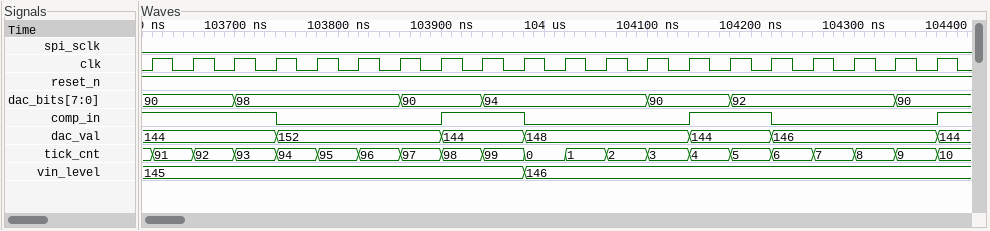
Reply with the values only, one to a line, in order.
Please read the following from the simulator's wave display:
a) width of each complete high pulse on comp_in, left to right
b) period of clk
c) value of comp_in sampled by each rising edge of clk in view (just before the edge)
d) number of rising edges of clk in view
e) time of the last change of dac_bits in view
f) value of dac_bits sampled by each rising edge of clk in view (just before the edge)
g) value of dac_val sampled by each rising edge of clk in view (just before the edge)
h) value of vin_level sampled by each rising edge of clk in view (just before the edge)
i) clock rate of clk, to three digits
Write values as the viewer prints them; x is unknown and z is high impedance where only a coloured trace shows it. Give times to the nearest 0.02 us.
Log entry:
0.08 us, 0.08 us
0.04 us
1 1 1 1 0 0 0 0 1 1 0 0 0 0 1 1 0 0 0 0
20
104.34 us
90, 90, 90, 98, 98, 98, 98, 90, 90, 94, 94, 94, 94, 90, 90, 92, 92, 92, 92, 90
144, 144, 144, 144, 152, 152, 152, 152, 144, 144, 148, 148, 148, 148, 144, 144, 146, 146, 146, 146
145, 145, 145, 145, 145, 145, 145, 145, 145, 145, 146, 146, 146, 146, 146, 146, 146, 146, 146, 146
25.0 MHz
